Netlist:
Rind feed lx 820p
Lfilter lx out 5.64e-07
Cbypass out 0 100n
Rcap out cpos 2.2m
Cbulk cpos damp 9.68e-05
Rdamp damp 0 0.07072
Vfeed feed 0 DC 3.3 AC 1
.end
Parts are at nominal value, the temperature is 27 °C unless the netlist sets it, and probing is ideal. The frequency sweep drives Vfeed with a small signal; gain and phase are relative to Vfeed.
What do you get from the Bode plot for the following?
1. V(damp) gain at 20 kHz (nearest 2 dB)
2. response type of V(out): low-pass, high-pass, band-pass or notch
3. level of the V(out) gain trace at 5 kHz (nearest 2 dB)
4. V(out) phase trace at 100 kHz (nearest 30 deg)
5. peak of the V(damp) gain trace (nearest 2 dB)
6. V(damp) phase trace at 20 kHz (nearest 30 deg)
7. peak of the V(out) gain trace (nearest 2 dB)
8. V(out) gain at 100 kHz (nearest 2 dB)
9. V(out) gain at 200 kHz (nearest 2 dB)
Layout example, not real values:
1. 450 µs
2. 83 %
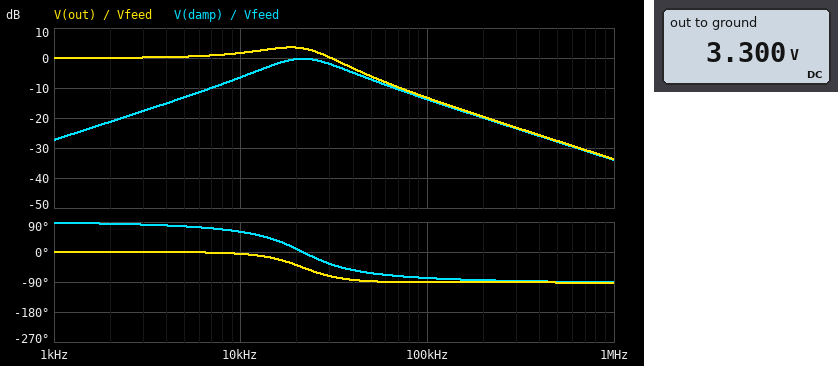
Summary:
1. 0 dB
2. low-pass
3. 0 dB
4. -90 deg
5. 0 dB
6. 0 deg
7. 4 dB
8. -14 dB
9. -20 dB
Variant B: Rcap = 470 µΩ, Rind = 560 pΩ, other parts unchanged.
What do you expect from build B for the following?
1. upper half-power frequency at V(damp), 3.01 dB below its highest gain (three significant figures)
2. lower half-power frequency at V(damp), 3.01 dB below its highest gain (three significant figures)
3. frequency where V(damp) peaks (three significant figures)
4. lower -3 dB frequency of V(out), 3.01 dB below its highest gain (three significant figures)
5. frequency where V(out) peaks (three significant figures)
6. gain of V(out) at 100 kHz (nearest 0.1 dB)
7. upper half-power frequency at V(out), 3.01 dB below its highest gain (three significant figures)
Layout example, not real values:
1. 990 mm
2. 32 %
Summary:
1. 33.8 kHz
2. 13.7 kHz
3. 21.5 kHz
4. 5.92 kHz
5. 18.7 kHz
6. -13.5 dB
7. 29.0 kHz
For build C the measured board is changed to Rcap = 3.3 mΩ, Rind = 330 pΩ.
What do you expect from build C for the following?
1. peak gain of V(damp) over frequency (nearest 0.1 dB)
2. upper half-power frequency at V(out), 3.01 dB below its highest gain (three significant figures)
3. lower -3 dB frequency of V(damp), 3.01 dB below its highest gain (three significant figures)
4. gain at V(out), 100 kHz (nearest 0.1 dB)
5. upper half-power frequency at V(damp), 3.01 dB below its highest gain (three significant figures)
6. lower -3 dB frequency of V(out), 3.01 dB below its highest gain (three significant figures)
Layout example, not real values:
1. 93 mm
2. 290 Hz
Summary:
1. -0.4 dB
2. 29.3 kHz
3. 13.5 kHz
4. -13.2 dB
5. 34.4 kHz
6. 5.04 kHz
